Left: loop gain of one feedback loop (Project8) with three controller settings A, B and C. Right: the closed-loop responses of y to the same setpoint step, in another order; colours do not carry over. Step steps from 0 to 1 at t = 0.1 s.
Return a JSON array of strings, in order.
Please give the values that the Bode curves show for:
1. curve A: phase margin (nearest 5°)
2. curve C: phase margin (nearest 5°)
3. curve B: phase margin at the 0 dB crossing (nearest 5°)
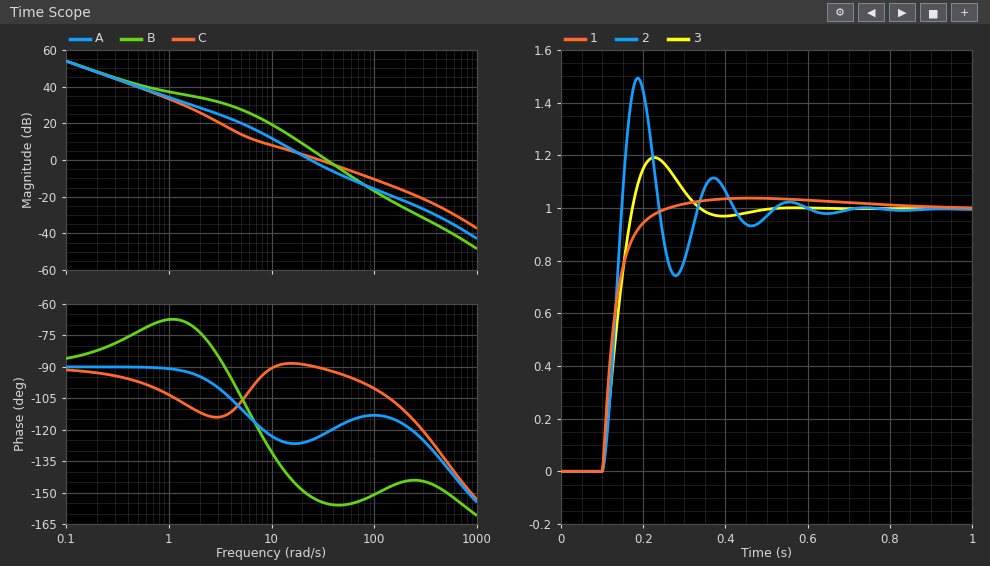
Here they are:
["55°", "90°", "25°"]
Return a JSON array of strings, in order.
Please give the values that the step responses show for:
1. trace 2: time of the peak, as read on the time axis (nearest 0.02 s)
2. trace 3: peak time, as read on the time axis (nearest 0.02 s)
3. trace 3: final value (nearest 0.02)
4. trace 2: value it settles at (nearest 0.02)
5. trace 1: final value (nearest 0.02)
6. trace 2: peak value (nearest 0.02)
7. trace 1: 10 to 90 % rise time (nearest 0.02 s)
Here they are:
["0.18 s", "0.22 s", "1.00", "1.00", "1.00", "1.50", "0.08 s"]
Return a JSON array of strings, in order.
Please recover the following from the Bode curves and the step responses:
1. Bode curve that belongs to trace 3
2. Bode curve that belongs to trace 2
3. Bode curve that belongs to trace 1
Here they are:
["A", "B", "C"]
